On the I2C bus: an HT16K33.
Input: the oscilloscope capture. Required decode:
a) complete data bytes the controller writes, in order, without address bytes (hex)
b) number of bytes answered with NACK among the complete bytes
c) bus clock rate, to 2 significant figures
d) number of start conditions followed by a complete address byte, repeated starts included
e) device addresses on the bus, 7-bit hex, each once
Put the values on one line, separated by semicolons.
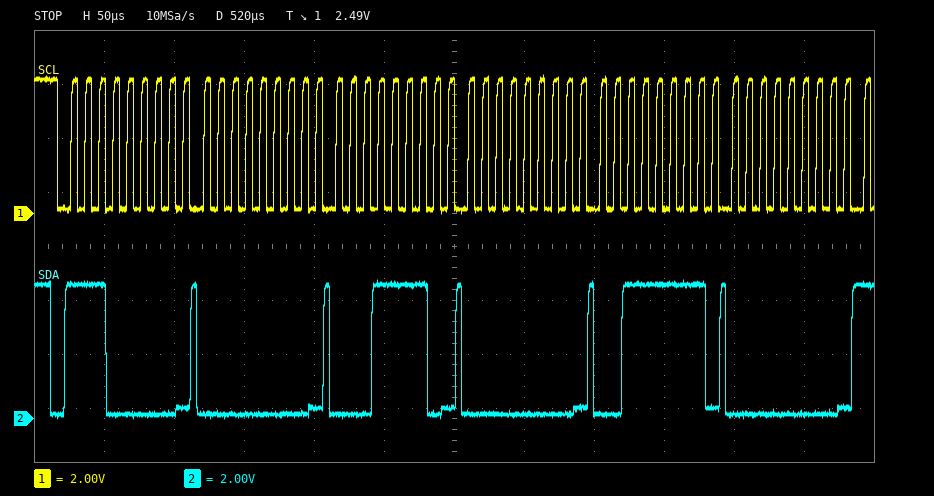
00 1E 00 3F 00; 0; 100 kHz; 1; 0x70
